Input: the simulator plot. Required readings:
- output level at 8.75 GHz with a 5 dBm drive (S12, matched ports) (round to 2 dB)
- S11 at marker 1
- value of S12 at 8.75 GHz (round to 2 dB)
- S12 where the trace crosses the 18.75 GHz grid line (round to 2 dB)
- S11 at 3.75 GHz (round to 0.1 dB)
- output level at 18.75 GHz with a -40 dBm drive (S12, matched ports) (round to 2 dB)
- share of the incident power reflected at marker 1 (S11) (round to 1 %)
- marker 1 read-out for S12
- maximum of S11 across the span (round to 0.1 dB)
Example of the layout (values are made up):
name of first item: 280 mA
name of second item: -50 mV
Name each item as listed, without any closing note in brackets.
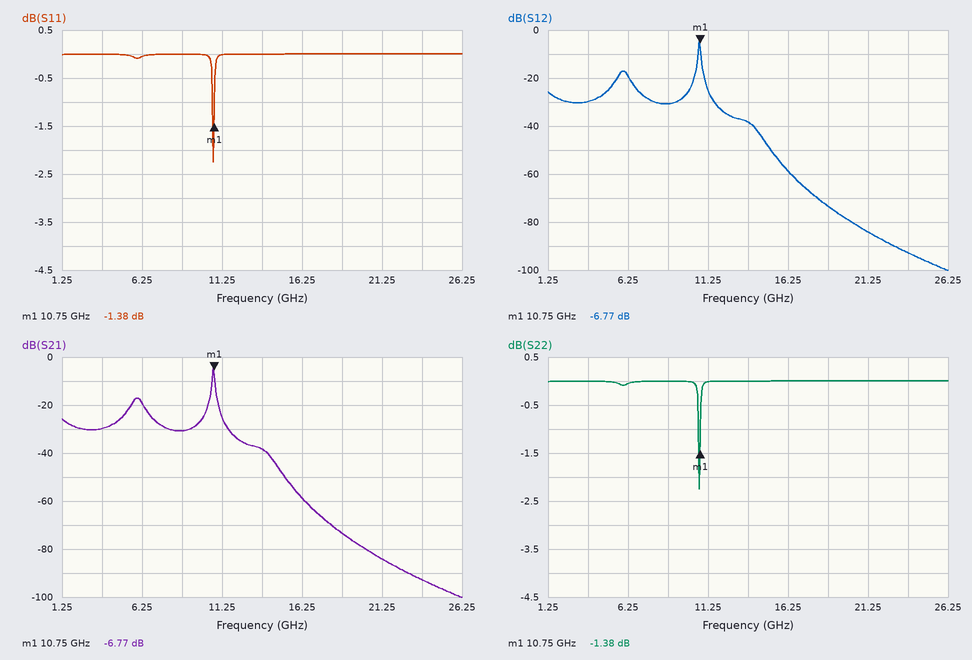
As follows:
output level at 8.75 GHz with a 5 dBm drive (S12, matched ports): -26 dBm
S11 at marker 1: -1.38 dB
value of S12 at 8.75 GHz: -30 dB
S12 where the trace crosses the 18.75 GHz grid line: -74 dB
S11 at 3.75 GHz: 0.0 dB
output level at 18.75 GHz with a -40 dBm drive (S12, matched ports): -114 dBm
share of the incident power reflected at marker 1 (S11): 73 %
marker 1 read-out for S12: -6.77 dB
maximum of S11 across the span: 0.0 dB
